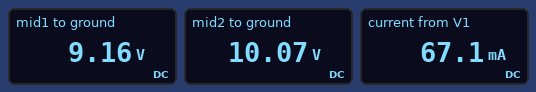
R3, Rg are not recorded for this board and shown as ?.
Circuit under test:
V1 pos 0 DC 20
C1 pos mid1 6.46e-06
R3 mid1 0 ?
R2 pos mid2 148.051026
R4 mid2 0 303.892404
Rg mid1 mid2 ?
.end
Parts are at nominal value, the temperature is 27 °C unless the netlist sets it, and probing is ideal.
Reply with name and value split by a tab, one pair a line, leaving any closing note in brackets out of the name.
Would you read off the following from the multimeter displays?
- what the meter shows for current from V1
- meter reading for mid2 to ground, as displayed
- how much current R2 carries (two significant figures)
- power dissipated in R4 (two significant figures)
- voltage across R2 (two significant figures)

what the meter shows for current from V1	67.1 mA
meter reading for mid2 to ground, as displayed	10.07 V
how much current R2 carries	67 mA
power dissipated in R4	330 mW
voltage across R2	9.9 V
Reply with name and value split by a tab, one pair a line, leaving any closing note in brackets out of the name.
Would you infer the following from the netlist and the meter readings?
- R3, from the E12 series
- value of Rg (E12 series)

R3, from the E12 series	270 Ω
value of Rg	27 Ω
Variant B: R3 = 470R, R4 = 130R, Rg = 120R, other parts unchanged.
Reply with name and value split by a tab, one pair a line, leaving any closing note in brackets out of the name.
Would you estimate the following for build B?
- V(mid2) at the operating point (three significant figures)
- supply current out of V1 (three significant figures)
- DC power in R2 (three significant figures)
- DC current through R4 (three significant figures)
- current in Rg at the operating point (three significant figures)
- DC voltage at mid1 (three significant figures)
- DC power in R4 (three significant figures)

V(mid2) at the operating point	8.37 V
supply current out of V1	78.6 mA
DC power in R2	914 mW
DC current through R4	64.4 mA
current in Rg at the operating point	14.2 mA
DC voltage at mid1	6.67 V
DC power in R4	539 mW
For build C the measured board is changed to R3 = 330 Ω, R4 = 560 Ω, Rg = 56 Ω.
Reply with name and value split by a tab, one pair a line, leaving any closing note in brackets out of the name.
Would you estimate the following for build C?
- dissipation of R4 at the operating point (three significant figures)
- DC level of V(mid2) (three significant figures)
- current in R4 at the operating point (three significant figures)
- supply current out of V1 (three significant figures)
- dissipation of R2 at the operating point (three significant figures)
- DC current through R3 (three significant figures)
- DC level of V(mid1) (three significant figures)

dissipation of R4 at the operating point	263 mW
DC level of V(mid2)	12.1 V
current in R4 at the operating point	21.7 mA
supply current out of V1	53.1 mA
dissipation of R2 at the operating point	418 mW
DC current through R3	31.4 mA
DC level of V(mid1)	10.4 V
